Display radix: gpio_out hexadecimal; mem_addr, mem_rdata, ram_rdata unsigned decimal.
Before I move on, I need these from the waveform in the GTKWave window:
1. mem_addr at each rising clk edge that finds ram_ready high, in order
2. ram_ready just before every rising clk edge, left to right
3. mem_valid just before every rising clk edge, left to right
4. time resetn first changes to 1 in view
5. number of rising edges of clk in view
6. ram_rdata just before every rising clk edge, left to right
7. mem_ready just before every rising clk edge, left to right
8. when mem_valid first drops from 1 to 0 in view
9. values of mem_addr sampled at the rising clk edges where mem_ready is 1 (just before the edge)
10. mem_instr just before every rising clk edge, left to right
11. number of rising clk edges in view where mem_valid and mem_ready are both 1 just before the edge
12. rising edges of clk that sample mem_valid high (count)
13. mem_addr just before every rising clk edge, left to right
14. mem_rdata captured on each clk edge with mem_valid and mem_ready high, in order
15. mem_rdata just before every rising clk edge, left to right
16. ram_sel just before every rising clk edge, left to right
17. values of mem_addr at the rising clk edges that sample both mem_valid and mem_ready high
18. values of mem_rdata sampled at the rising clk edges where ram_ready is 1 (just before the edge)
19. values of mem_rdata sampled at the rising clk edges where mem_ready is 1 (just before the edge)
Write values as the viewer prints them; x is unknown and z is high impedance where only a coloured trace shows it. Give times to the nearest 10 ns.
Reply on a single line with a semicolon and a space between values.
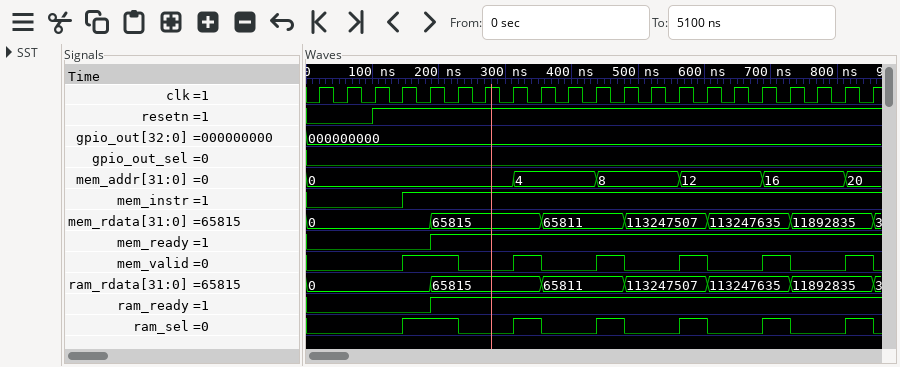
0, 0, 0, 4, 4, 4, 8, 8, 8, 12, 12, 12, 16, 16, 16, 20; 0 0 0 0 0 1 1 1 1 1 1 1 1 1 1 1 1 1 1 1 1; 0 0 0 0 1 1 0 0 1 0 0 1 0 0 1 0 0 1 0 0 1; 100 ns; 21; 0, 0, 0, 0, 0, 65815, 65815, 65815, 65815, 65811, 65811, 65811, 113247507, 113247507, 113247507, 113247635, 113247635, 113247635, 11892835, 11892835, 11892835; 0 0 0 0 0 1 1 1 1 1 1 1 1 1 1 1 1 1 1 1 1; 230 ns; 0, 0, 0, 4, 4, 4, 8, 8, 8, 12, 12, 12, 16, 16, 16, 20; 0 0 0 0 1 1 1 1 1 1 1 1 1 1 1 1 1 1 1 1 1; 6; 7; 0, 0, 0, 0, 0, 0, 0, 0, 4, 4, 4, 8, 8, 8, 12, 12, 12, 16, 16, 16, 20; 65815, 65815, 65811, 113247507, 113247635, 11892835; 0, 0, 0, 0, 0, 65815, 65815, 65815, 65815, 65811, 65811, 65811, 113247507, 113247507, 113247507, 113247635, 113247635, 113247635, 11892835, 11892835, 11892835; 0 0 0 0 1 1 0 0 1 0 0 1 0 0 1 0 0 1 0 0 1; 0, 4, 8, 12, 16, 20; 65815, 65815, 65815, 65815, 65811, 65811, 65811, 113247507, 113247507, 113247507, 113247635, 113247635, 113247635, 11892835, 11892835, 11892835; 65815, 65815, 65815, 65815, 65811, 65811, 65811, 113247507, 113247507, 113247507, 113247635, 113247635, 113247635, 11892835, 11892835, 11892835
